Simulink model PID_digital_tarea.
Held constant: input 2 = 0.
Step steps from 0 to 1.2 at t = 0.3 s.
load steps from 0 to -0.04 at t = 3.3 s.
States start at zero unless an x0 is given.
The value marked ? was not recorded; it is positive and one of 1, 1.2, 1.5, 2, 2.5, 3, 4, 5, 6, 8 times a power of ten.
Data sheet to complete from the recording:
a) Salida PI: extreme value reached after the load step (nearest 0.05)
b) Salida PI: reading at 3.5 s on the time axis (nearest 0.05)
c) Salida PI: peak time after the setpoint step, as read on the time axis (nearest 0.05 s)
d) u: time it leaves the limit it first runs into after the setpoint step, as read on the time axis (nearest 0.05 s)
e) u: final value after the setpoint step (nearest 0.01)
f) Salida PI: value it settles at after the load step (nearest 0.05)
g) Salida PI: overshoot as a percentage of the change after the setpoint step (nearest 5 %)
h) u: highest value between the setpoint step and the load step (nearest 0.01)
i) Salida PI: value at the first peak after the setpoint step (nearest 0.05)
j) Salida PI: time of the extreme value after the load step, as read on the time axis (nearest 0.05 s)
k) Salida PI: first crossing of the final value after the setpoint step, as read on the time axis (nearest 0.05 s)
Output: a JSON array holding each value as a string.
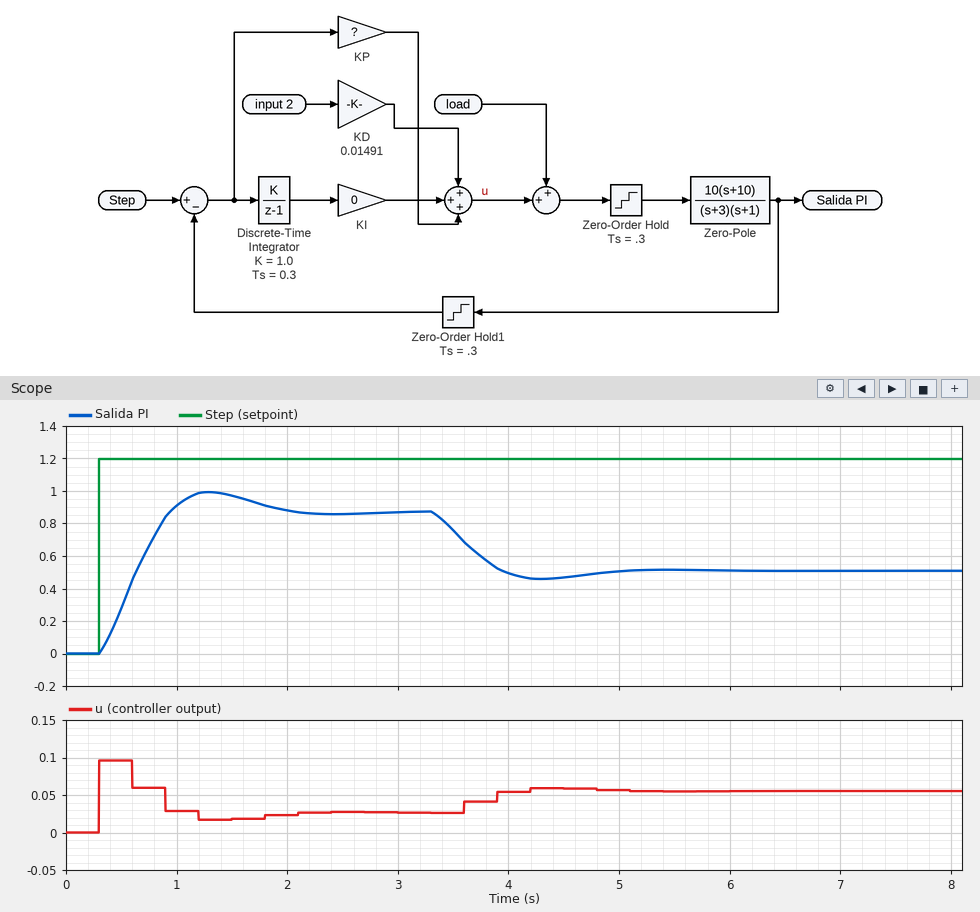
["0.45", "0.75", "1.30 s", "0.60 s", "0.03", "0.50", "15 %", "0.10", "1.00", "4.30 s", "0.95 s"]
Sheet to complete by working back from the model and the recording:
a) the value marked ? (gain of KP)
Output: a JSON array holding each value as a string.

["0.08"]
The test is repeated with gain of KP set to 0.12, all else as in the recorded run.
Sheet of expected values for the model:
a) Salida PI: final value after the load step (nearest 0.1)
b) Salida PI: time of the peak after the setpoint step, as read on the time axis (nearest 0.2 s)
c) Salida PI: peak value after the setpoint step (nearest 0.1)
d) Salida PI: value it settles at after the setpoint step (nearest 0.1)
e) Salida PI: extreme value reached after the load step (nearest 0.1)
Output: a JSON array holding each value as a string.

["0.7", "1.0 s", "1.2", "1.0", "0.6"]
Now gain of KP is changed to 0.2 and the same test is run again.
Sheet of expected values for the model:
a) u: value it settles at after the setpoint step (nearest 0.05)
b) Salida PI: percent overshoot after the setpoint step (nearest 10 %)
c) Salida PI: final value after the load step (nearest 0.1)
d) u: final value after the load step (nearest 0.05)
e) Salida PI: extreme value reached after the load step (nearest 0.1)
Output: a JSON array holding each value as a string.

["0.05", "40 %", "0.9", "0.05", "0.8"]
